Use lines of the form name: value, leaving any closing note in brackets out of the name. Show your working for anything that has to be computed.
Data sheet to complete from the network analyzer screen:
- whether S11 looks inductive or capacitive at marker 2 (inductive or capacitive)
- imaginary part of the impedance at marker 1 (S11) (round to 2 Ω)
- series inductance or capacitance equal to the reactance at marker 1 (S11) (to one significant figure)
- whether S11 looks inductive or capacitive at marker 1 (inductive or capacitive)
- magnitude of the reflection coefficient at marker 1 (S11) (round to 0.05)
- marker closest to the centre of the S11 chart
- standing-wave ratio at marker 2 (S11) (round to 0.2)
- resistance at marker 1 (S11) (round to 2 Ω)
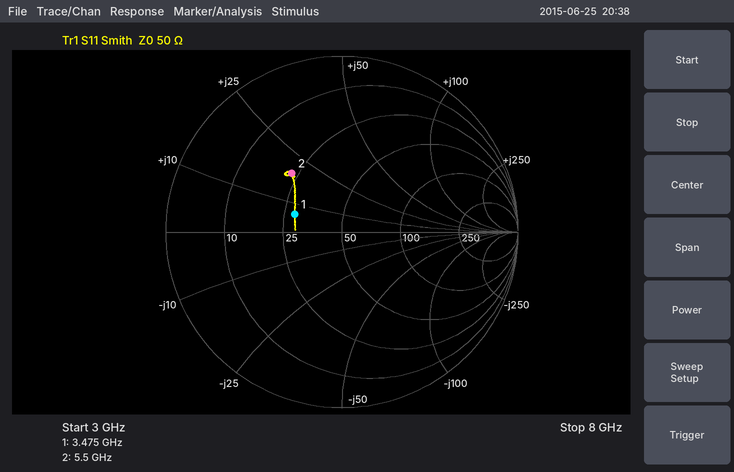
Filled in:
whether S11 looks inductive or capacitive at marker 2: inductive
imaginary part of the impedance at marker 1 (S11): +6 Ω
series inductance or capacitance equal to the reactance at marker 1 (S11): L = 6 Ω/(2π × 3.475 GHz) ≈ 275 pH, so 300 pH to one significant figure
whether S11 looks inductive or capacitive at marker 1: inductive
magnitude of the reflection coefficient at marker 1 (S11): 0.30
marker closest to the centre of the S11 chart: marker 1
standing-wave ratio at marker 2 (S11): 2.6
resistance at marker 1 (S11): 28 Ω
